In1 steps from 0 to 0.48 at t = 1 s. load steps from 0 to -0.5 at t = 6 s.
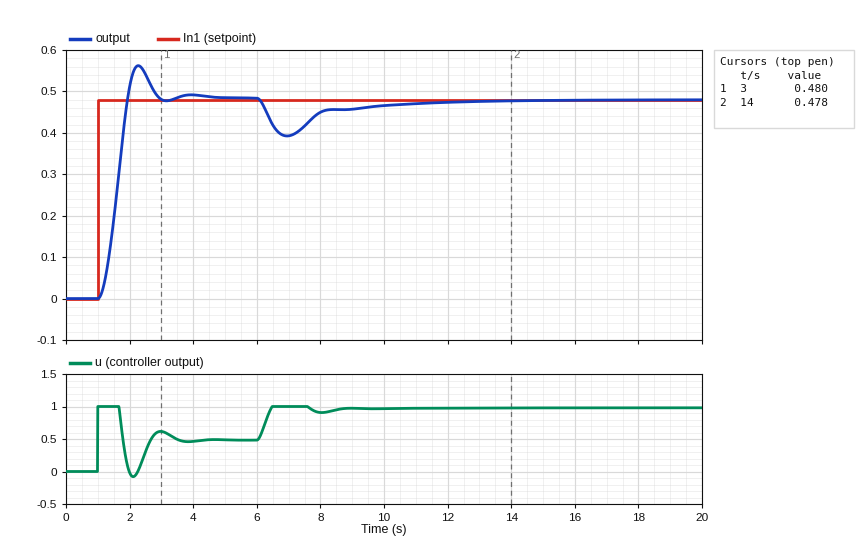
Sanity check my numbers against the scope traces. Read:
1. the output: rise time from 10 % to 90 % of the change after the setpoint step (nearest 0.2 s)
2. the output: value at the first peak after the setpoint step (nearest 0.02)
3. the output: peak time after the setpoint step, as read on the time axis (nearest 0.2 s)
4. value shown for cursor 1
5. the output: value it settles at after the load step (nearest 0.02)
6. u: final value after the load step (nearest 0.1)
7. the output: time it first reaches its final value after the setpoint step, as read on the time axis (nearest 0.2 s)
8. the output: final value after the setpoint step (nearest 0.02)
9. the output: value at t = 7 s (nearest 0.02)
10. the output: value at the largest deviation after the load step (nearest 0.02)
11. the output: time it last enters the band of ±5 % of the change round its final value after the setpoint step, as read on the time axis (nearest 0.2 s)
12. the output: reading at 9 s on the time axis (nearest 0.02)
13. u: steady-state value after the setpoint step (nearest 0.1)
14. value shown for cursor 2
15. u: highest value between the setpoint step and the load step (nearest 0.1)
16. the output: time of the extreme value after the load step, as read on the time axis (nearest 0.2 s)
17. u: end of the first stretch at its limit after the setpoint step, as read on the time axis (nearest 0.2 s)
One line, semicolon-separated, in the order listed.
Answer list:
0.6 s; 0.56; 2.2 s; 0.480; 0.48; 1.0; 2.0 s; 0.48; 0.40; 0.40; 2.8 s; 0.46; 0.5; 0.478; 1.0; 7.0 s; 1.6 s
